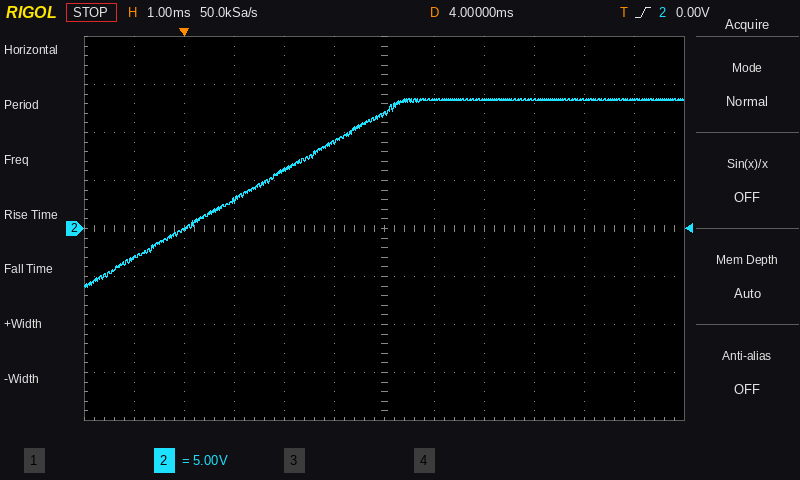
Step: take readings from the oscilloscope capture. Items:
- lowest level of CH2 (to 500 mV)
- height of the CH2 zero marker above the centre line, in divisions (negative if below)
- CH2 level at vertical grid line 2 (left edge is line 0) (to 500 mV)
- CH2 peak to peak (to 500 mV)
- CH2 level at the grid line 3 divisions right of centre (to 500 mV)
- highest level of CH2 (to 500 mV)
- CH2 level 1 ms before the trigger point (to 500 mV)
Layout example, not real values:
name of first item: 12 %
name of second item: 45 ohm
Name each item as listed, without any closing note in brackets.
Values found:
lowest level of CH2: -6.0 V
height of the CH2 zero marker above the centre line, in divisions: 0.0 div
CH2 level at vertical grid line 2 (left edge is line 0): 0.0 V
CH2 peak to peak: 19.5 V
CH2 level at the grid line 3 divisions right of centre: 13.5 V
highest level of CH2: 13.5 V
CH2 level 1 ms before the trigger point: -3.0 V
